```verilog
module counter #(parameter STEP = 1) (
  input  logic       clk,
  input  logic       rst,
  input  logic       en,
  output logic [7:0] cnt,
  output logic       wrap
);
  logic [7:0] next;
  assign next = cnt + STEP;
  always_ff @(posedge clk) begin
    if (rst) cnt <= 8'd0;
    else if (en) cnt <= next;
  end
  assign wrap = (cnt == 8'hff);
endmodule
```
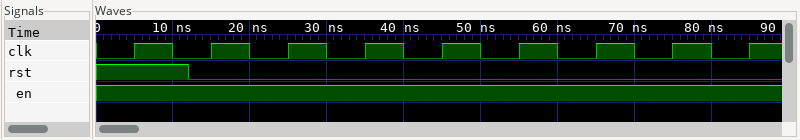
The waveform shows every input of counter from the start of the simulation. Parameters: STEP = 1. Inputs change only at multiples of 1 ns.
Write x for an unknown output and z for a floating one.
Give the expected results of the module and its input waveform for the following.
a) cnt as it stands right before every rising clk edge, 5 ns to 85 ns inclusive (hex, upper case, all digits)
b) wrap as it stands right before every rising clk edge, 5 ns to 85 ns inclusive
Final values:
x, 00, 01, 02, 03, 04, 05, 06, 07
x 0 0 0 0 0 0 0 0
